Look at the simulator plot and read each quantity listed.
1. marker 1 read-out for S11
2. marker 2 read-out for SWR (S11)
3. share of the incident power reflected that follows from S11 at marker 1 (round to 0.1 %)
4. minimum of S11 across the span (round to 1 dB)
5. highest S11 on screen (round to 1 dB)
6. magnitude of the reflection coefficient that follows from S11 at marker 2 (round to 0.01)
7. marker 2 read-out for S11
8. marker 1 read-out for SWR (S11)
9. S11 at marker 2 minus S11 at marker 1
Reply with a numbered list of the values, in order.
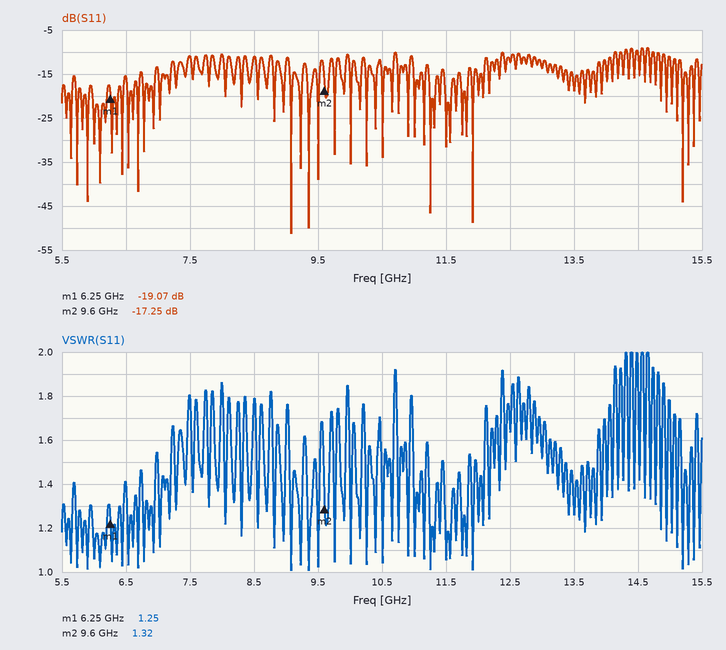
1. -19.07 dB
2. 1.32
3. 1.2 %
4. -51 dB
5. -9 dB
6. 0.14
7. -17.25 dB
8. 1.25
9. 1.82 dB
